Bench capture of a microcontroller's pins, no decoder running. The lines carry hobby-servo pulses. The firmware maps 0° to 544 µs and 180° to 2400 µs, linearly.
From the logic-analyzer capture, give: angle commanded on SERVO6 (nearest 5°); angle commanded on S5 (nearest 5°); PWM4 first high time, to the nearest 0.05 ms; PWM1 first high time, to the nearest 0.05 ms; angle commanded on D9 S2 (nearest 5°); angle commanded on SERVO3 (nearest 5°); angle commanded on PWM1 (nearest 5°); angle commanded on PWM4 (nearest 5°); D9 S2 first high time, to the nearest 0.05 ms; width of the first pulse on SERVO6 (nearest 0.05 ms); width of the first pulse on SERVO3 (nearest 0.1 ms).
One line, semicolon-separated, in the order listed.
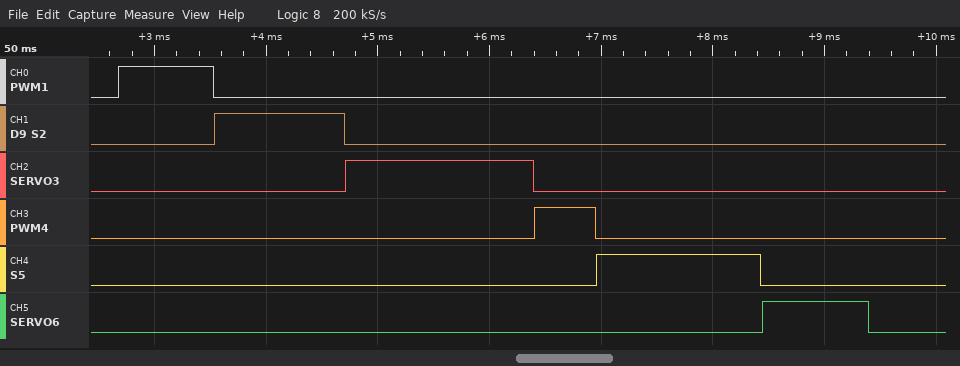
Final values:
40°; 90°; 0.55 ms; 0.85 ms; 60°; 110°; 30°; 0°; 1.15 ms; 0.95 ms; 1.7 ms
